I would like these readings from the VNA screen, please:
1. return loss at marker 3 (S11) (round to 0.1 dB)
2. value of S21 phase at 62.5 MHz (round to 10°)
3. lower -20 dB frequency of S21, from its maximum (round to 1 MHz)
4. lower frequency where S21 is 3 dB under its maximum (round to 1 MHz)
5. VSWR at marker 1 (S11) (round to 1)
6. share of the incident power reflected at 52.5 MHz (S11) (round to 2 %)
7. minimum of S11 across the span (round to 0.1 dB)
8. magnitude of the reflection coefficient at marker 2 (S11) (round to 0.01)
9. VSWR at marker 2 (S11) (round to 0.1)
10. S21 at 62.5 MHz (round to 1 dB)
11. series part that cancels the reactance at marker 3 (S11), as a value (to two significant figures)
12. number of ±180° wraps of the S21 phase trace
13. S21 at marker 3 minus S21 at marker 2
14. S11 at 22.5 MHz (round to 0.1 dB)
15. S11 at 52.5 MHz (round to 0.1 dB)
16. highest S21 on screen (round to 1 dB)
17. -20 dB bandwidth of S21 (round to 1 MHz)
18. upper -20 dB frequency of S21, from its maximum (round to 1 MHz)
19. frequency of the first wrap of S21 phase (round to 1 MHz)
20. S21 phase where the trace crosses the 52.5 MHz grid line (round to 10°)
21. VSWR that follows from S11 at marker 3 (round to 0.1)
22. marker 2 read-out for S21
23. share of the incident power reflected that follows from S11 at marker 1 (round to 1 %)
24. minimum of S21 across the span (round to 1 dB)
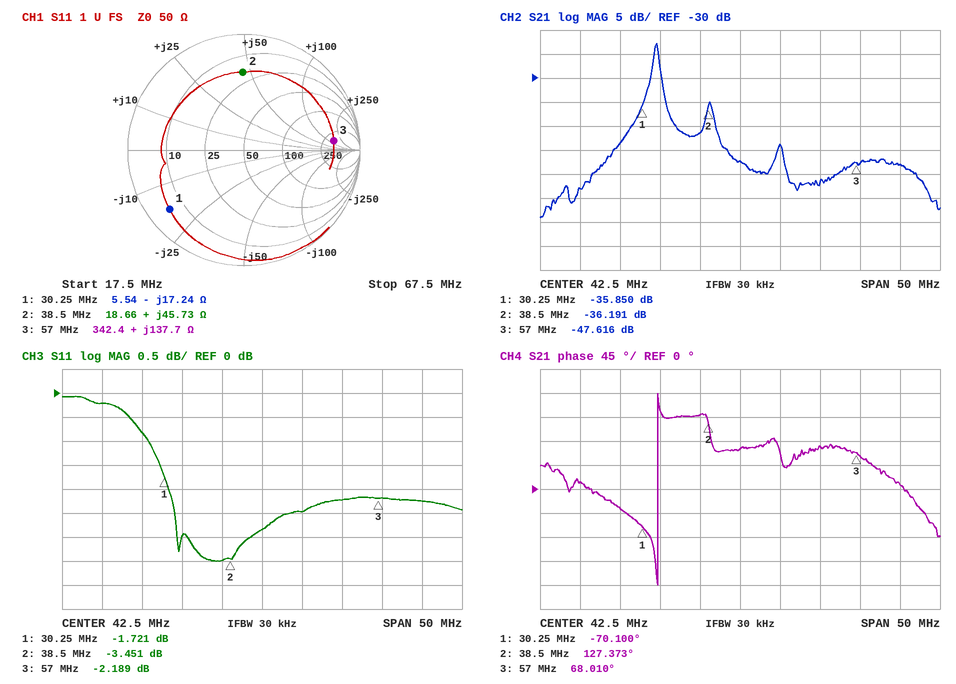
2.2 dB
10°
28 MHz
32 MHz
10
60 %
-3.5 dB
0.67
5.1
-48 dB
20 pF
1
-11.425 dB
-0.2 dB
-2.2 dB
-23 dB
12 MHz
40 MHz
32 MHz
80°
8.0
-36.191 dB
67 %
-59 dB
